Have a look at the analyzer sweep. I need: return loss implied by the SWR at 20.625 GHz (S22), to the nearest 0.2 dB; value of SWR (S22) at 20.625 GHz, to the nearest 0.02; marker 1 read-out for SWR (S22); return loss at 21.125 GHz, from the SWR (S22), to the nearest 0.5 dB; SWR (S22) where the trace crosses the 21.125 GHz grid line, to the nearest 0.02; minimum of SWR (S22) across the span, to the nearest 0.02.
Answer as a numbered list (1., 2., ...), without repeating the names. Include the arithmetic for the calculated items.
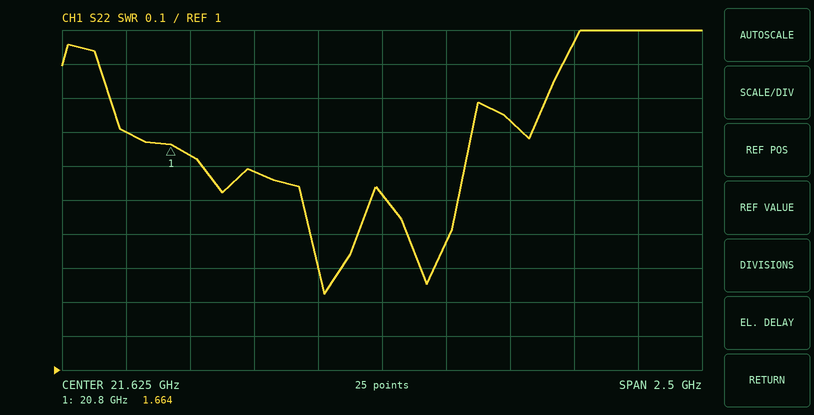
1. −20 log10((1.7 − 1)/(1.7 + 1)) ≈ 11.7 dB, so 11.8 dB to the nearest 0.2 dB
2. 1.70
3. 1.664
4. −20 log10((1.58 − 1)/(1.58 + 1)) ≈ 13.0 dB
5. 1.58
6. 1.22
